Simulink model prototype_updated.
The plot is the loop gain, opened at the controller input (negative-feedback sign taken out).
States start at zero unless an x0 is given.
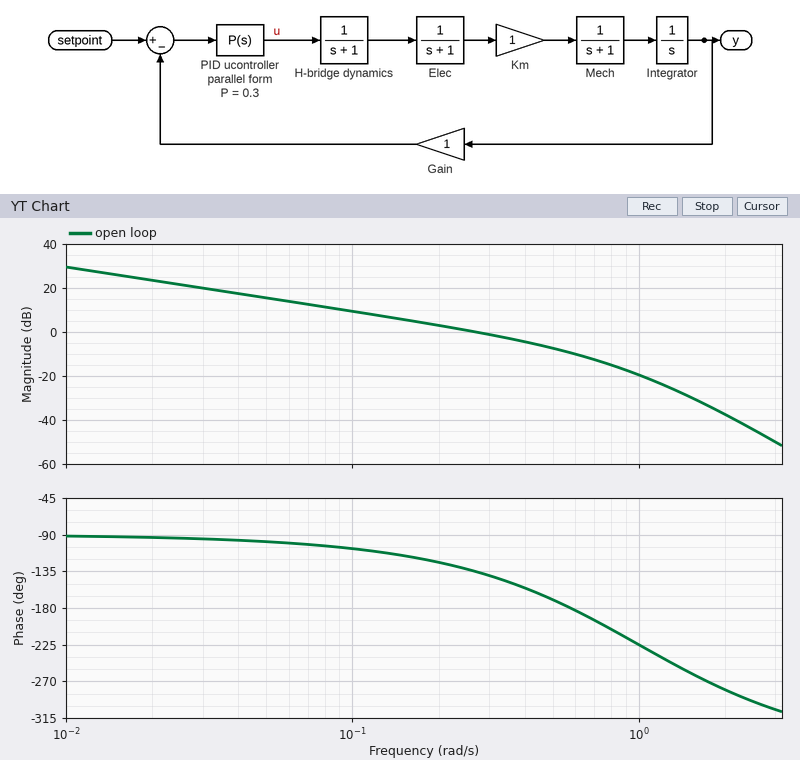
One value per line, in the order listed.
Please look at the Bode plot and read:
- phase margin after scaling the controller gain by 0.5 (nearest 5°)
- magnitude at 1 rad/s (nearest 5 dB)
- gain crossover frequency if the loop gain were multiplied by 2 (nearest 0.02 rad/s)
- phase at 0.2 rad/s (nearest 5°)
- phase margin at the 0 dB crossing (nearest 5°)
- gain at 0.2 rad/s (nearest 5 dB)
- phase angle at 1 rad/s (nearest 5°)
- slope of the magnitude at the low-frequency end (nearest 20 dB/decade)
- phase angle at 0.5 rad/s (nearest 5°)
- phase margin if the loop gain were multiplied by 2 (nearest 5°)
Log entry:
65°
-20 dB
0.46 rad/s
-125°
45°
5 dB
-225°
-20 dB/decade
-170°
15°
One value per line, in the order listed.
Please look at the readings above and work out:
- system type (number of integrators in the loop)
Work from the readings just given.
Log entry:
1
